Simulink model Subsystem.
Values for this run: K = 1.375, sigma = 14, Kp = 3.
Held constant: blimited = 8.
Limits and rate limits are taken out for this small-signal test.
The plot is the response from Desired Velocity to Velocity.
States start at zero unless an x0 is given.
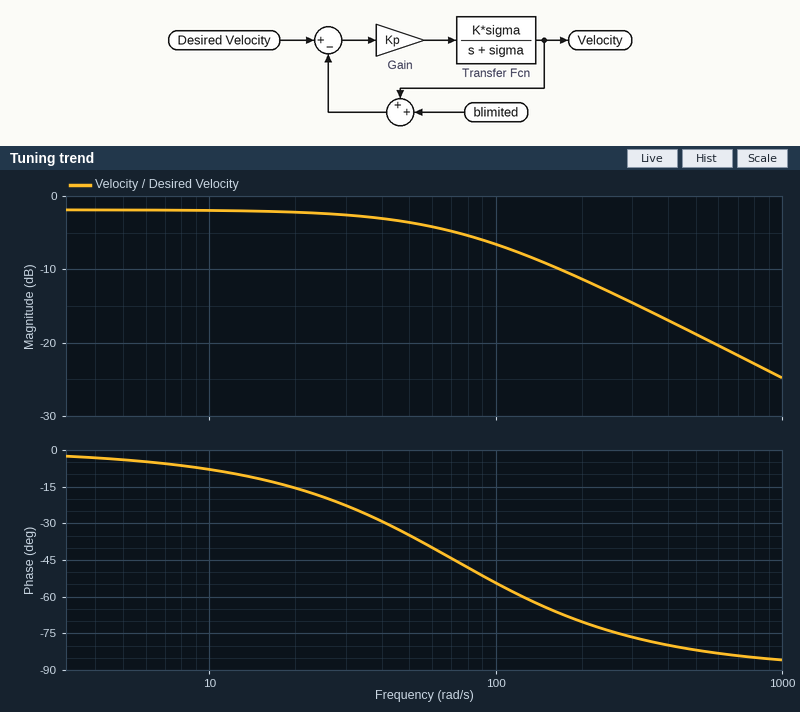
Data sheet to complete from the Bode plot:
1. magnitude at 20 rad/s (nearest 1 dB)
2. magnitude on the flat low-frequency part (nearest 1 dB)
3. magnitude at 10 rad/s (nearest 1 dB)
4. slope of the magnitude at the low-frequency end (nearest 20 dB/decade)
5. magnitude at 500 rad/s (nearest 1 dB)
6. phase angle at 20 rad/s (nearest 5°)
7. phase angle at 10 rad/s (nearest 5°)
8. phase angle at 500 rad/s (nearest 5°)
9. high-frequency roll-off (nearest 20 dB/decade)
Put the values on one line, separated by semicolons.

-2 dB; -2 dB; -2 dB; 0 dB/decade; -19 dB; -15°; -10°; -80°; -20 dB/decade
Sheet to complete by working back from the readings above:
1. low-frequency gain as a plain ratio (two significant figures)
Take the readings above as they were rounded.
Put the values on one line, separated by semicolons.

0.79
